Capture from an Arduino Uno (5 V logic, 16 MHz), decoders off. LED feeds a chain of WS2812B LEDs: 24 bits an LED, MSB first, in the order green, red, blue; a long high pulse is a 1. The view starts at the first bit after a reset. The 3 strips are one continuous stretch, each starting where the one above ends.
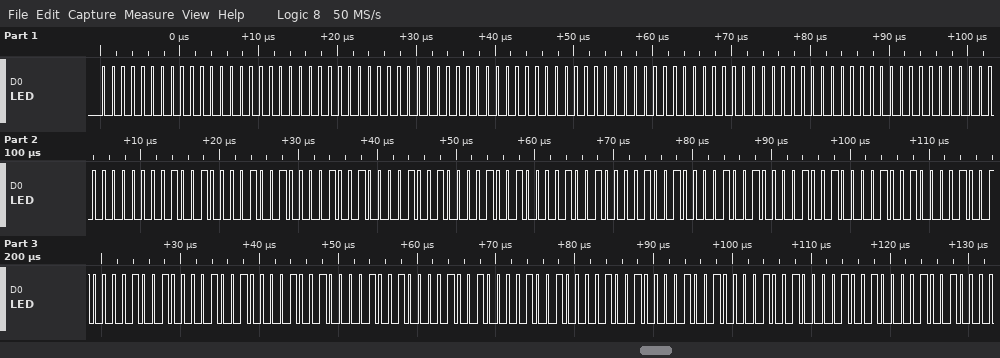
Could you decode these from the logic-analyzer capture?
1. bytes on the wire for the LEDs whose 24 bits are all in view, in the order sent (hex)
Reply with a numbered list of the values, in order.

1. 00 00 00 00 00 00 00 00 00 00 00 00 12 12 12 12 12 12 12 12 12 12 12 12 12 12 12 12 12 12 12 12 12
